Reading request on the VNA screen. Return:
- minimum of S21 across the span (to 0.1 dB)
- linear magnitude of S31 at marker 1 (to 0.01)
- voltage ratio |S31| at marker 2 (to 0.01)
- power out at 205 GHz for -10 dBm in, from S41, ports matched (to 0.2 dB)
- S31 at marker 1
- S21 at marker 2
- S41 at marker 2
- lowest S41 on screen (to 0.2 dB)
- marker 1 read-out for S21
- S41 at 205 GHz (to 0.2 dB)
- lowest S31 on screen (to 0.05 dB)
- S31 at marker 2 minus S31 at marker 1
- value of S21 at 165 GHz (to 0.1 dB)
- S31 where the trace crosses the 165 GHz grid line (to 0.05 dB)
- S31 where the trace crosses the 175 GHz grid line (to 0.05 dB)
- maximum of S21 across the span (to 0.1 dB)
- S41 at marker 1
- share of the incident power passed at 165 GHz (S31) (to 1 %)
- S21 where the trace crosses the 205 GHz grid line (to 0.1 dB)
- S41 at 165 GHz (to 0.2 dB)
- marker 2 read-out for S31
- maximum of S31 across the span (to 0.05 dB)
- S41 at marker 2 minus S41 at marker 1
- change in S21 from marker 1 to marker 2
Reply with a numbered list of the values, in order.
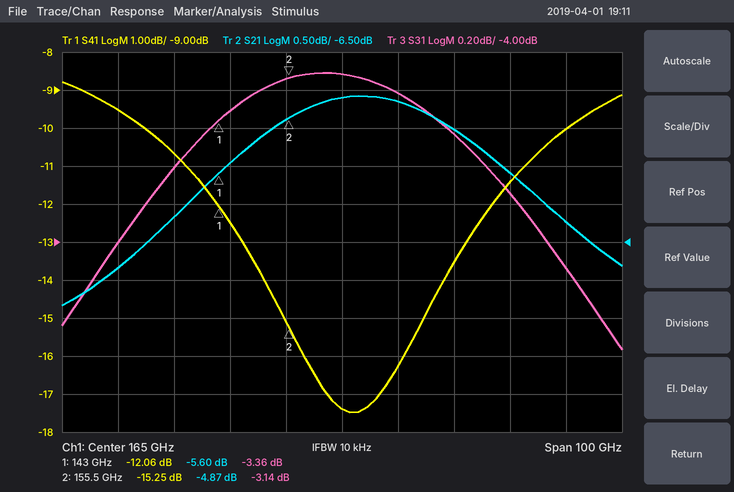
1. -7.3 dB
2. 0.68
3. 0.70
4. -20.0 dBm
5. -3.36 dB
6. -4.87 dB
7. -15.25 dB
8. -17.4 dB
9. -5.60 dB
10. -10.0 dB
11. -4.55 dB
12. 0.22 dB
13. -4.6 dB
14. -3.10 dB
15. -3.20 dB
16. -4.6 dB
17. -12.06 dB
18. 49 %
19. -6.2 dB
20. -17.4 dB
21. -3.14 dB
22. -3.10 dB
23. -3.19 dB
24. 0.73 dB
